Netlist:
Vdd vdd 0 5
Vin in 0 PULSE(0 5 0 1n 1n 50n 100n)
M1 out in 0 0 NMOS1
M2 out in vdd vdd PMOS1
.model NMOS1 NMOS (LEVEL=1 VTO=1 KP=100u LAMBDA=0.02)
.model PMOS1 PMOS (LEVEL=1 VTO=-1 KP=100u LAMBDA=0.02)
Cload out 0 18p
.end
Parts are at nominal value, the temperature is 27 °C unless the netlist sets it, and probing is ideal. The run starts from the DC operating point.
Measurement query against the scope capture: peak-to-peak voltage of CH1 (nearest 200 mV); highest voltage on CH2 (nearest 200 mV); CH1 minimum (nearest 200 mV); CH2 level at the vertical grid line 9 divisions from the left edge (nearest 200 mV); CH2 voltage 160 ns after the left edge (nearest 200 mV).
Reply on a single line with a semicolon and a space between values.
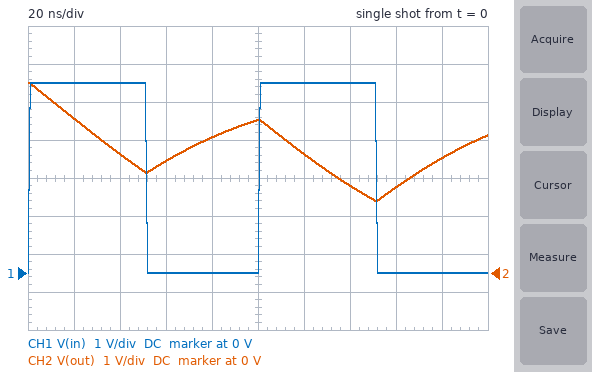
5.0 V; 5.0 V; 0 V; 3.0 V; 2.2 V
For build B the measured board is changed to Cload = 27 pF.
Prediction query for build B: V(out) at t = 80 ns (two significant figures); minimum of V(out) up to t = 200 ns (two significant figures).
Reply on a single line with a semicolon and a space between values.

3.9 V; 2.6 V
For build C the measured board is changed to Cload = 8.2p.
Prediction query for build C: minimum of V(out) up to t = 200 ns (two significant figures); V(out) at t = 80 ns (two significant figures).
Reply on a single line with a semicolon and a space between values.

660 mV; 3.4 V
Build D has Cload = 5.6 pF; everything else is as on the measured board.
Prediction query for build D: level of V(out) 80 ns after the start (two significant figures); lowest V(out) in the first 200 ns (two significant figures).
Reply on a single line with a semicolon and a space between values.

3.8 V; 260 mV
